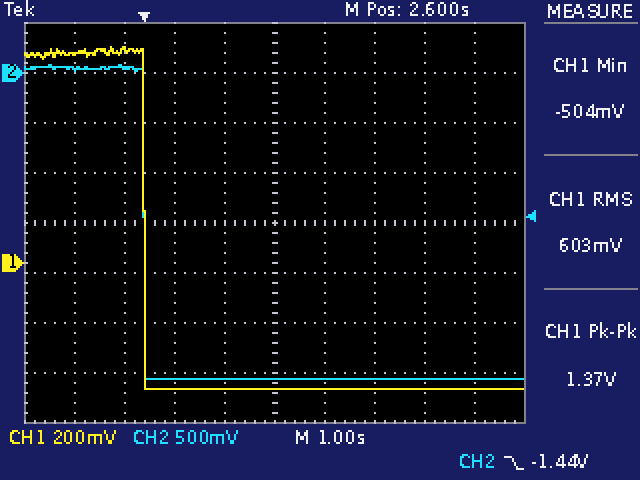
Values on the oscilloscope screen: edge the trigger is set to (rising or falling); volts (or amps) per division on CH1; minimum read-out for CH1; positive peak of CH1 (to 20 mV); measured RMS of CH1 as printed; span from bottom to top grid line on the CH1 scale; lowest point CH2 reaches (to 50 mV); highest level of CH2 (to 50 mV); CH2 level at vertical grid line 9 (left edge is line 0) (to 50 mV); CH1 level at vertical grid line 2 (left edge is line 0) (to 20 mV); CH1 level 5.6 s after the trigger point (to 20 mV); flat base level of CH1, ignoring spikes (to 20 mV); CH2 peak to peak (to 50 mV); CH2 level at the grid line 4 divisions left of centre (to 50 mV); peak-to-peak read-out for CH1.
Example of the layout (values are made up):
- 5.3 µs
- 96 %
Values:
- falling
- 200 mV
- -504 mV
- 860 mV
- 603 mV
- 1.6 V
- -3.05 V
- 100 mV
- -3.05 V
- 860 mV
- -500 mV
- -500 mV
- 3.15 V
- 50 mV
- 1.37 V
